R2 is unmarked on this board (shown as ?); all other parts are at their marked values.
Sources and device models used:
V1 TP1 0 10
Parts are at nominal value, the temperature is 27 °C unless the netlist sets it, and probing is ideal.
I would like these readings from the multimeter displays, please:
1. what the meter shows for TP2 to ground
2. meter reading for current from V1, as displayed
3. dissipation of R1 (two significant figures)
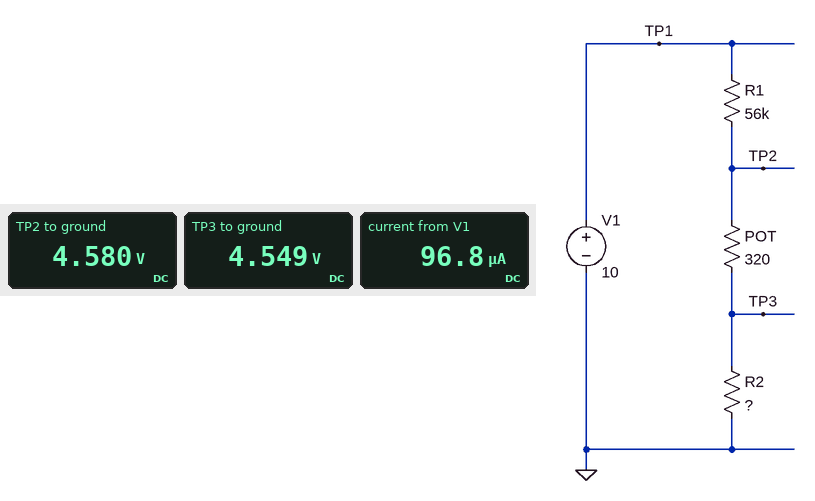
4.580 V
96.8 µA
520 µW
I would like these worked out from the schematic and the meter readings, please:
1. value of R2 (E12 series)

47 kΩ
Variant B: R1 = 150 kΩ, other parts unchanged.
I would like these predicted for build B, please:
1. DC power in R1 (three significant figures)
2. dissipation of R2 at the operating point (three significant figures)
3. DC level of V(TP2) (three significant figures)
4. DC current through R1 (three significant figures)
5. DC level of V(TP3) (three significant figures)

385 µW
121 µW
2.40 V
50.7 µA
2.38 V
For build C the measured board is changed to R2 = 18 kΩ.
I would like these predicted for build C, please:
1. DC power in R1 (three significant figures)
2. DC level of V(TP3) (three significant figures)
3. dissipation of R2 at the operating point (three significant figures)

1.01 mW
2.42 V
326 µW
